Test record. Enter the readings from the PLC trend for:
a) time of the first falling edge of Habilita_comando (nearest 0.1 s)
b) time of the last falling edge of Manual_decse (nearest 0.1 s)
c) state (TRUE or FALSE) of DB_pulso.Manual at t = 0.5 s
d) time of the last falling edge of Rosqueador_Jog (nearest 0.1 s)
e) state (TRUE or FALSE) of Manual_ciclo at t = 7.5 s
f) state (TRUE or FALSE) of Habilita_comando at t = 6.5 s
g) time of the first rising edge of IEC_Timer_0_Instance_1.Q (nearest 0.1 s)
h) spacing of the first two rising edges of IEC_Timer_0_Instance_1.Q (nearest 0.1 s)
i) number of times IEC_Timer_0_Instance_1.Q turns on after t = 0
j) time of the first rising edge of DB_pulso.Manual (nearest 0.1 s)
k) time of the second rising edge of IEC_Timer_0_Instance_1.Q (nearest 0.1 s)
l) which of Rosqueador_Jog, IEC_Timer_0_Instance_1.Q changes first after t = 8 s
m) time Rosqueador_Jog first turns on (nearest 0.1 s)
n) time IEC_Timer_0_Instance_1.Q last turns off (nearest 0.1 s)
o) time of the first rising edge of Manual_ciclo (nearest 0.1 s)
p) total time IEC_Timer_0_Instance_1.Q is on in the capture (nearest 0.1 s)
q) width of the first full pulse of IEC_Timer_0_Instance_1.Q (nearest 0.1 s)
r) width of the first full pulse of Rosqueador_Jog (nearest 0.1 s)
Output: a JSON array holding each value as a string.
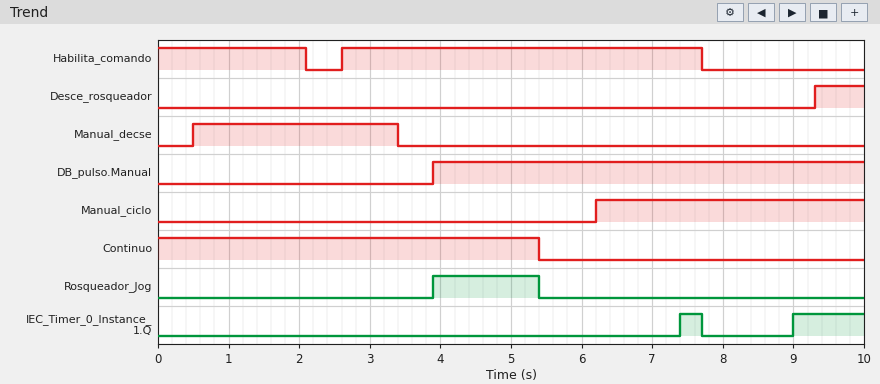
["2.1 s", "3.4 s", "FALSE", "5.4 s", "TRUE", "TRUE", "7.4 s", "1.6 s", "2", "3.9 s", "9.0 s", "IEC_Timer_0_Instance_1.Q", "3.9 s", "7.7 s", "6.2 s", "1.3 s", "0.3 s", "1.5 s"]
